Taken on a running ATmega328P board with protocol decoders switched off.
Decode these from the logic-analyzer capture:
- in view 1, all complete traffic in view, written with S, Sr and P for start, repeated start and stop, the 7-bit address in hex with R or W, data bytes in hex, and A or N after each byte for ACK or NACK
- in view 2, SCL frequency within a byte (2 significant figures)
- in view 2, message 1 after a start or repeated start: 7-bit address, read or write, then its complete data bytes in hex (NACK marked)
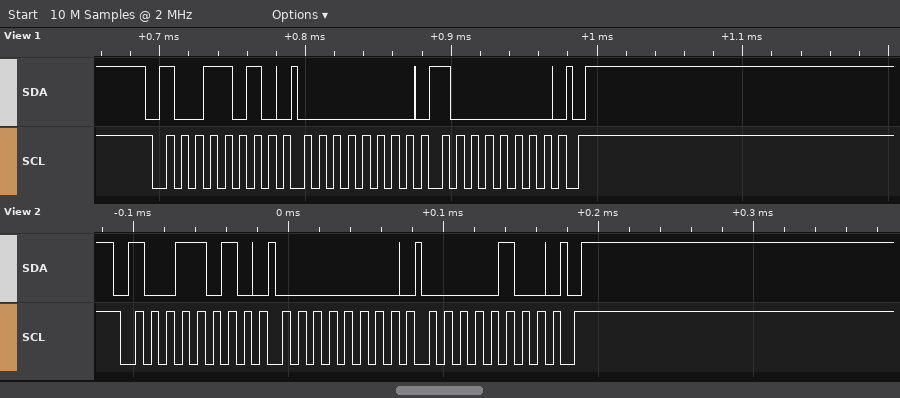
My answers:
S 4DW A 00 A 80 A P
100 kHz
0x4D write: 00 04
